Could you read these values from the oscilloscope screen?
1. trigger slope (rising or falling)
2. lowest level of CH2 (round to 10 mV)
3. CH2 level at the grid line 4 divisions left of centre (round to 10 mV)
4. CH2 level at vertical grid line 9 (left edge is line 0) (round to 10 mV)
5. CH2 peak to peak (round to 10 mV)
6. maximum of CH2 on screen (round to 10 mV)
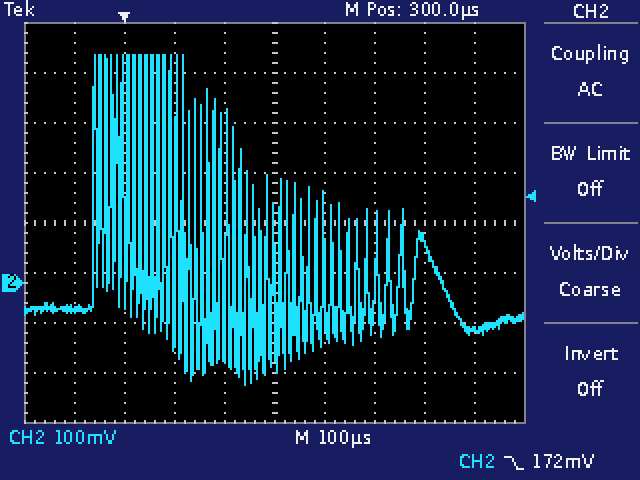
falling
-200 mV
-50 mV
-90 mV
660 mV
460 mV
